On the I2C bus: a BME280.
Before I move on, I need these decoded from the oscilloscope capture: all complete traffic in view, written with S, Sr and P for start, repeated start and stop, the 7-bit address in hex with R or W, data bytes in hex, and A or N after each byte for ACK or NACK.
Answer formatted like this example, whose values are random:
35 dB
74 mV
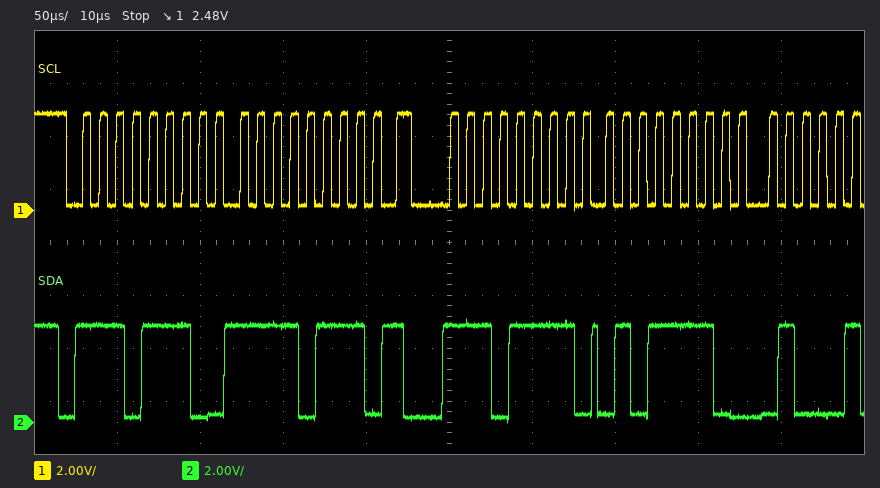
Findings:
S 77W A F7 A Sr 77R A 5E A
